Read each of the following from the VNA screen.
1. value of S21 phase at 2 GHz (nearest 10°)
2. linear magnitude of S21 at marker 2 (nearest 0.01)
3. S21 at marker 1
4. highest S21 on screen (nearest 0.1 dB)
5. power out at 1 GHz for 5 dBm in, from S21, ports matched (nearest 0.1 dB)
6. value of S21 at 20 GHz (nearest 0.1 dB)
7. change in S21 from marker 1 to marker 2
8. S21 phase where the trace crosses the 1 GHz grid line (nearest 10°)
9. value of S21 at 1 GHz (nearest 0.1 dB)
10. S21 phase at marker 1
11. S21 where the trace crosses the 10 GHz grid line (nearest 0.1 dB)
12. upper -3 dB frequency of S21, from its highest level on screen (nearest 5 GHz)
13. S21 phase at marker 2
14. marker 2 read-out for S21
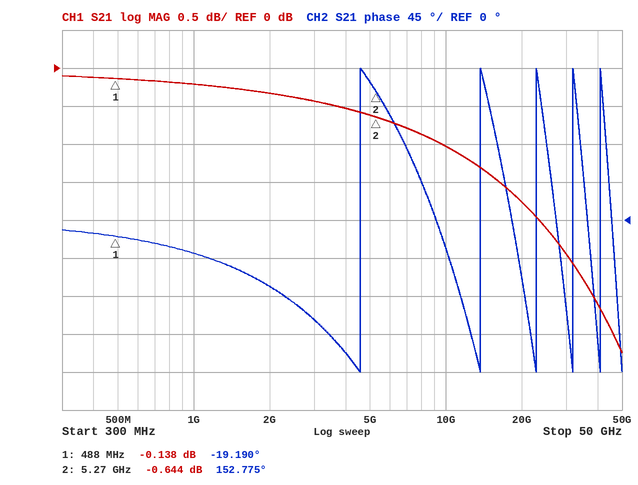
-80°
0.93
-0.138 dB
-0.1 dB
4.8 dBm
-1.8 dB
-0.506 dB
-40°
-0.2 dB
-19.190°
-1.0 dB
40 GHz
152.775°
-0.644 dB
